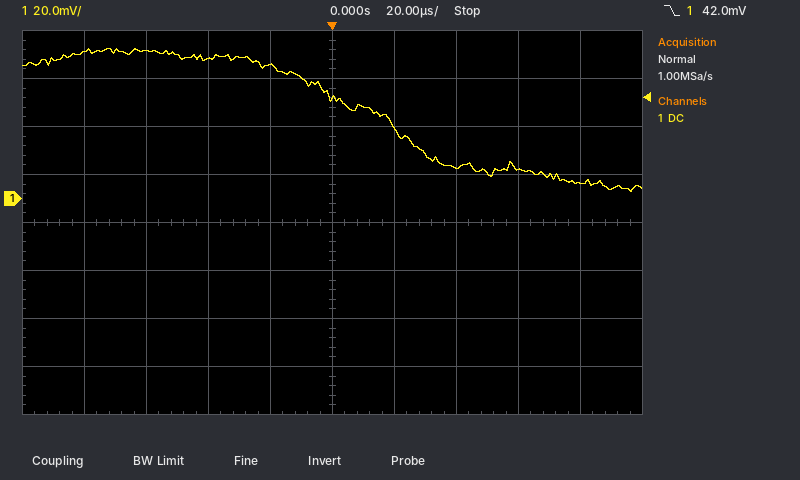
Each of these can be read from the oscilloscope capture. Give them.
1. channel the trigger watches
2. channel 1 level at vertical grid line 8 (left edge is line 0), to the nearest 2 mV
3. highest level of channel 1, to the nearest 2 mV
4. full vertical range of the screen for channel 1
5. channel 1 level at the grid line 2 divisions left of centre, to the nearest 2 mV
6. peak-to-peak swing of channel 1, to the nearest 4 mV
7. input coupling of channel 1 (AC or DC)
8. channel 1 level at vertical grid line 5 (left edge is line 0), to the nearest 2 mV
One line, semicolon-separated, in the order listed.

channel 1; 12 mV; 62 mV; 160 mV; 58 mV; 60 mV; DC; 42 mV
